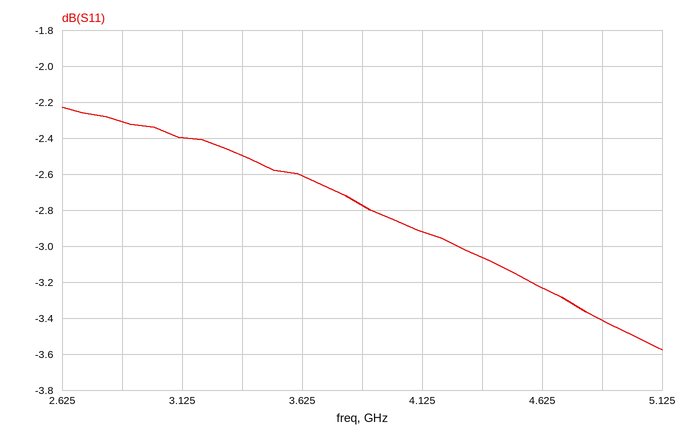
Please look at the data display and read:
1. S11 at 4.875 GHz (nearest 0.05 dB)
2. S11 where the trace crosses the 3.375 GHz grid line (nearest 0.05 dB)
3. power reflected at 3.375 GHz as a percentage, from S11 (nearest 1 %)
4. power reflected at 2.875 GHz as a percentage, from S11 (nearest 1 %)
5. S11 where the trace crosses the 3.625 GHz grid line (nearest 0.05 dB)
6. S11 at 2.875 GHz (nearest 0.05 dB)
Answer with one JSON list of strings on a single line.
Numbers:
["-3.40 dB", "-2.50 dB", "56 %", "59 %", "-2.60 dB", "-2.30 dB"]
